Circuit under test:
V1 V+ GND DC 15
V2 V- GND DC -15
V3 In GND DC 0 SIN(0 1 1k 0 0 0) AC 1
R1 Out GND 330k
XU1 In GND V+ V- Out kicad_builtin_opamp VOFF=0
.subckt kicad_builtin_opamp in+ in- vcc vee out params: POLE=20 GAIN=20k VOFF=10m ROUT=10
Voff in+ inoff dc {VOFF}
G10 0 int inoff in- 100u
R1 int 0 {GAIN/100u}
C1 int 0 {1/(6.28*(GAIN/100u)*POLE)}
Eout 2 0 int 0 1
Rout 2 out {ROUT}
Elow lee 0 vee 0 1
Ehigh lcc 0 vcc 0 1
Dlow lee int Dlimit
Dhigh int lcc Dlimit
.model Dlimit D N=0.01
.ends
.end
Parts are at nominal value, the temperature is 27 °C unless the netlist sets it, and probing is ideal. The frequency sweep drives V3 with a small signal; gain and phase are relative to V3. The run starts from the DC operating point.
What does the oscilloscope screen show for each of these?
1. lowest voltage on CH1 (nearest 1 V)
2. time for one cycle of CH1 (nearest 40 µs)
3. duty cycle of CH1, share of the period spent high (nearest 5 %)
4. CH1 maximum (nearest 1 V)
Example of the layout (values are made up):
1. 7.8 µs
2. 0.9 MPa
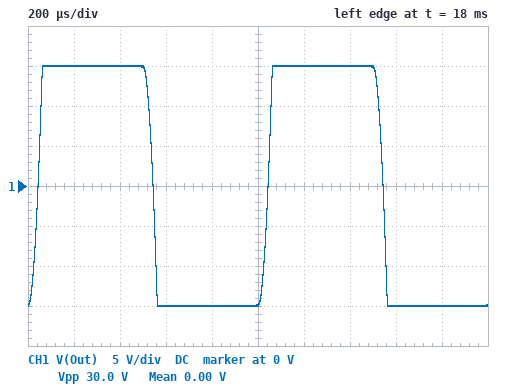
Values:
1. -15 V
2. 1.00 ms
3. 50 %
4. 15 V
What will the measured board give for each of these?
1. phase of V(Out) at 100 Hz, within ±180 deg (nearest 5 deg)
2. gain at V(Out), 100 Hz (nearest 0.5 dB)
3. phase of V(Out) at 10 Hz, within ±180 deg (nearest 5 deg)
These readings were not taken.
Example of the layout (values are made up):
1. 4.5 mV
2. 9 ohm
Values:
1. -80 deg
2. 72.0 dB
3. -25 deg
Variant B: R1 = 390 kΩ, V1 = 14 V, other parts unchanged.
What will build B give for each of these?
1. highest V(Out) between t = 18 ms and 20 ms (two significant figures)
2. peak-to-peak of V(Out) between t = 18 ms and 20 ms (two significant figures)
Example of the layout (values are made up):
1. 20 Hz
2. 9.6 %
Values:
1. 14 V
2. 29 V
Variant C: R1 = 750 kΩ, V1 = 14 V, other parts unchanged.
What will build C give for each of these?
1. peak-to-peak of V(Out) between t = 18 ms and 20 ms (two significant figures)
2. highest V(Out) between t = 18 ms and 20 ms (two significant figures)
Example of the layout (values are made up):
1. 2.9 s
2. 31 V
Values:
1. 29 V
2. 14 V
